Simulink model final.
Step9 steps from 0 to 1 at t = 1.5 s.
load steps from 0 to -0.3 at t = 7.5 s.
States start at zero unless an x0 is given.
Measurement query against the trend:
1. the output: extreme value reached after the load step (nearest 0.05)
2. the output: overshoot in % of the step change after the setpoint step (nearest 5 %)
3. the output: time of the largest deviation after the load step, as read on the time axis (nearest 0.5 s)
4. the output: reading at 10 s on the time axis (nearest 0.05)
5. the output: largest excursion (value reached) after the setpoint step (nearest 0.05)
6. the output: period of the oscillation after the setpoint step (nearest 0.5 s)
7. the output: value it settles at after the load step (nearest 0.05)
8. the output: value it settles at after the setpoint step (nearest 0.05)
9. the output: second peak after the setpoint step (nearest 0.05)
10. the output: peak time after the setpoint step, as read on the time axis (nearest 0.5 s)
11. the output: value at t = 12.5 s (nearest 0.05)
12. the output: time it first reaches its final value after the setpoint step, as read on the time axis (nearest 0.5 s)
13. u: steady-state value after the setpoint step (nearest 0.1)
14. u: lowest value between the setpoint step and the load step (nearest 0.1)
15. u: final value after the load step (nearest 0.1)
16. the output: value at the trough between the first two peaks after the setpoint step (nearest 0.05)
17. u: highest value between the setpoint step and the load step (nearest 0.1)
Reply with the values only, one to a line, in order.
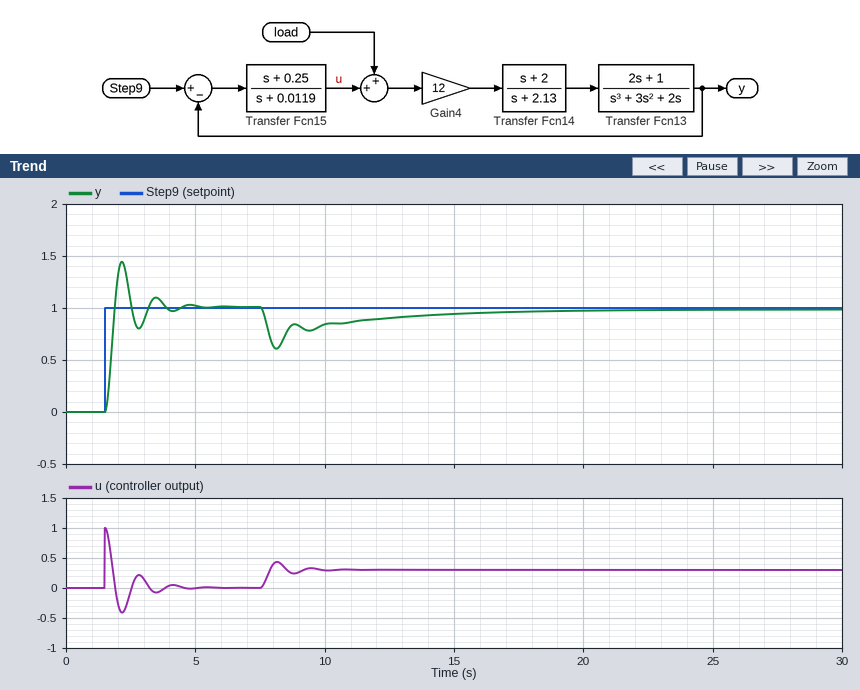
0.60
45 %
8.0 s
0.85
1.45
1.5 s
1.00
1.00
1.10
2.0 s
0.90
2.0 s
0.0
-0.4
0.3
0.80
1.0
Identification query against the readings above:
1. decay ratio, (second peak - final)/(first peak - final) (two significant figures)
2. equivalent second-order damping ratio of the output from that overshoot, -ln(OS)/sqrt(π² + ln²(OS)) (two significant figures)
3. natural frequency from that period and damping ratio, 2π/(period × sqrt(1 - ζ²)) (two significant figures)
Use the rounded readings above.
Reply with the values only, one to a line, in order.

0.22
0.25
4.3 rad/s
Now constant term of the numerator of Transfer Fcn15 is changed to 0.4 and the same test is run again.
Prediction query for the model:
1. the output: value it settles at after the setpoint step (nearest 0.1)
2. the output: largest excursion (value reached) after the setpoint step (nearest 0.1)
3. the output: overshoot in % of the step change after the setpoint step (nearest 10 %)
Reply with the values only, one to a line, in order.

1.0
1.5
50 %
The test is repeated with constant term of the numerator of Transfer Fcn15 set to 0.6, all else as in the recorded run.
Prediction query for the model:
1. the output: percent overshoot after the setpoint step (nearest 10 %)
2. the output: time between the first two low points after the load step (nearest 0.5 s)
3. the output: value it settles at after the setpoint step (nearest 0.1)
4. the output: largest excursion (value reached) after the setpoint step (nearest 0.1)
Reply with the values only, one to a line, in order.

50 %
1.5 s
1.0
1.5
